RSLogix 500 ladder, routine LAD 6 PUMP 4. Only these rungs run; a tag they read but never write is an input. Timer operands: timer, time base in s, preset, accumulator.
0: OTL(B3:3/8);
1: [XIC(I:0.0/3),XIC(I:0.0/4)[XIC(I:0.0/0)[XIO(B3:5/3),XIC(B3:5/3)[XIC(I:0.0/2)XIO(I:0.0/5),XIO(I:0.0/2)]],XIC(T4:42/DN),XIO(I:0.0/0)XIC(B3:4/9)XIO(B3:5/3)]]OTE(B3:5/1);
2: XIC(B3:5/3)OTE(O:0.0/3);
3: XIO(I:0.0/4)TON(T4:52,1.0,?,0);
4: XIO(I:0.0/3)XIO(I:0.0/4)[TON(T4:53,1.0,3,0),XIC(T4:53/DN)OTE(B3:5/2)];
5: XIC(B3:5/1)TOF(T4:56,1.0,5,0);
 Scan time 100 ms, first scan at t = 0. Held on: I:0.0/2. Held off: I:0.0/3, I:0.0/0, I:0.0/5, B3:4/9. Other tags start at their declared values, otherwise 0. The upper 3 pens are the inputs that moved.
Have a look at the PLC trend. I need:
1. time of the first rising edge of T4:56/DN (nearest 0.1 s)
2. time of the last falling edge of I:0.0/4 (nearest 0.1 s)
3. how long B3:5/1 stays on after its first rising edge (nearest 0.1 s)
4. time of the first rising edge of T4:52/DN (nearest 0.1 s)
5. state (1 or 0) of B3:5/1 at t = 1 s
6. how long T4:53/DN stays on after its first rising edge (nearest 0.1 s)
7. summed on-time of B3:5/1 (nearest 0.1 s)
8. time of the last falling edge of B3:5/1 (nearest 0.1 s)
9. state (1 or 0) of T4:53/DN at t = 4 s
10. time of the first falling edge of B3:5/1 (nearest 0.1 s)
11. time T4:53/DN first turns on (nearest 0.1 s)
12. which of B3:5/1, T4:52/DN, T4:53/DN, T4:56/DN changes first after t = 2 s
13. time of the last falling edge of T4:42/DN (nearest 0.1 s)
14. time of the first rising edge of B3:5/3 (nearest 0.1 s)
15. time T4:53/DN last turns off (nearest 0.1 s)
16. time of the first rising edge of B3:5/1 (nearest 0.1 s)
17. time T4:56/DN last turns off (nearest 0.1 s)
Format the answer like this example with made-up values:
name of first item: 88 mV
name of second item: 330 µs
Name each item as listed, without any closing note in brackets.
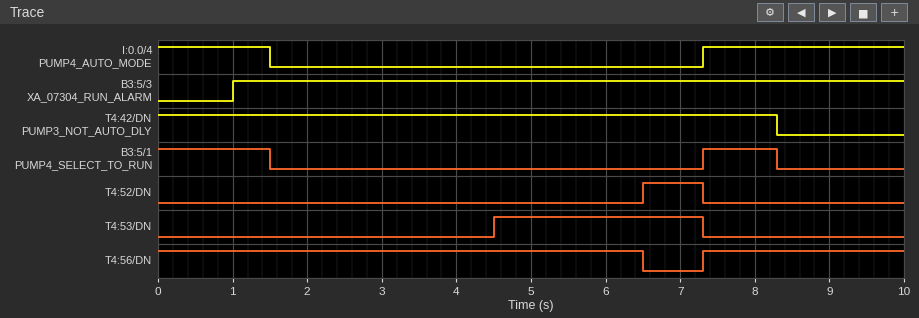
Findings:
time of the first rising edge of T4:56/DN: 7.3 s
time of the last falling edge of I:0.0/4: 1.5 s
how long B3:5/1 stays on after its first rising edge: 1.0 s
time of the first rising edge of T4:52/DN: 6.5 s
state (1 or 0) of B3:5/1 at t = 1 s: 1
how long T4:53/DN stays on after its first rising edge: 2.8 s
summed on-time of B3:5/1: 2.5 s
time of the last falling edge of B3:5/1: 8.3 s
state (1 or 0) of T4:53/DN at t = 4 s: 0
time of the first falling edge of B3:5/1: 1.5 s
time T4:53/DN first turns on: 4.5 s
which of B3:5/1, T4:52/DN, T4:53/DN, T4:56/DN changes first after t = 2 s: T4:53/DN
time of the last falling edge of T4:42/DN: 8.3 s
time of the first rising edge of B3:5/3: 1.0 s
time T4:53/DN last turns off: 7.3 s
time of the first rising edge of B3:5/1: 7.3 s
time T4:56/DN last turns off: 6.5 s
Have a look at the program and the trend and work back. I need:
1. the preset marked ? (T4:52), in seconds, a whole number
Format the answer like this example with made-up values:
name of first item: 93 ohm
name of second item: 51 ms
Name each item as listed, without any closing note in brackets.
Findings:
the preset marked ? (T4:52), in seconds, a whole number: 5 s
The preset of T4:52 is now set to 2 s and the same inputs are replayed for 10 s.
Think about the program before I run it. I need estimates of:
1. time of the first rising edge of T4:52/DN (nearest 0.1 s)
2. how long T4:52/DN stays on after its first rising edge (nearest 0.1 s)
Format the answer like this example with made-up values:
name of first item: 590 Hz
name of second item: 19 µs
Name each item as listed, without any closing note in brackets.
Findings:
time of the first rising edge of T4:52/DN: 3.5 s
how long T4:52/DN stays on after its first rising edge: 3.8 s
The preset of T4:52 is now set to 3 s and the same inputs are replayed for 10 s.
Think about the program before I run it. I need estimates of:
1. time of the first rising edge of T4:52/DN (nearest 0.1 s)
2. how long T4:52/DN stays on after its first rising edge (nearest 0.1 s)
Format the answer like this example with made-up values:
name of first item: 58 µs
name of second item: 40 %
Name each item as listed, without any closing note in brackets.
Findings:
time of the first rising edge of T4:52/DN: 4.5 s
how long T4:52/DN stays on after its first rising edge: 2.8 s
